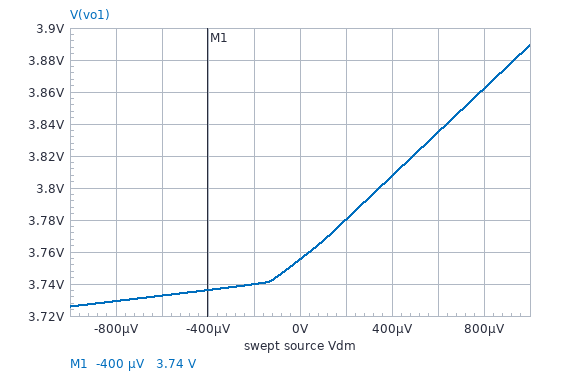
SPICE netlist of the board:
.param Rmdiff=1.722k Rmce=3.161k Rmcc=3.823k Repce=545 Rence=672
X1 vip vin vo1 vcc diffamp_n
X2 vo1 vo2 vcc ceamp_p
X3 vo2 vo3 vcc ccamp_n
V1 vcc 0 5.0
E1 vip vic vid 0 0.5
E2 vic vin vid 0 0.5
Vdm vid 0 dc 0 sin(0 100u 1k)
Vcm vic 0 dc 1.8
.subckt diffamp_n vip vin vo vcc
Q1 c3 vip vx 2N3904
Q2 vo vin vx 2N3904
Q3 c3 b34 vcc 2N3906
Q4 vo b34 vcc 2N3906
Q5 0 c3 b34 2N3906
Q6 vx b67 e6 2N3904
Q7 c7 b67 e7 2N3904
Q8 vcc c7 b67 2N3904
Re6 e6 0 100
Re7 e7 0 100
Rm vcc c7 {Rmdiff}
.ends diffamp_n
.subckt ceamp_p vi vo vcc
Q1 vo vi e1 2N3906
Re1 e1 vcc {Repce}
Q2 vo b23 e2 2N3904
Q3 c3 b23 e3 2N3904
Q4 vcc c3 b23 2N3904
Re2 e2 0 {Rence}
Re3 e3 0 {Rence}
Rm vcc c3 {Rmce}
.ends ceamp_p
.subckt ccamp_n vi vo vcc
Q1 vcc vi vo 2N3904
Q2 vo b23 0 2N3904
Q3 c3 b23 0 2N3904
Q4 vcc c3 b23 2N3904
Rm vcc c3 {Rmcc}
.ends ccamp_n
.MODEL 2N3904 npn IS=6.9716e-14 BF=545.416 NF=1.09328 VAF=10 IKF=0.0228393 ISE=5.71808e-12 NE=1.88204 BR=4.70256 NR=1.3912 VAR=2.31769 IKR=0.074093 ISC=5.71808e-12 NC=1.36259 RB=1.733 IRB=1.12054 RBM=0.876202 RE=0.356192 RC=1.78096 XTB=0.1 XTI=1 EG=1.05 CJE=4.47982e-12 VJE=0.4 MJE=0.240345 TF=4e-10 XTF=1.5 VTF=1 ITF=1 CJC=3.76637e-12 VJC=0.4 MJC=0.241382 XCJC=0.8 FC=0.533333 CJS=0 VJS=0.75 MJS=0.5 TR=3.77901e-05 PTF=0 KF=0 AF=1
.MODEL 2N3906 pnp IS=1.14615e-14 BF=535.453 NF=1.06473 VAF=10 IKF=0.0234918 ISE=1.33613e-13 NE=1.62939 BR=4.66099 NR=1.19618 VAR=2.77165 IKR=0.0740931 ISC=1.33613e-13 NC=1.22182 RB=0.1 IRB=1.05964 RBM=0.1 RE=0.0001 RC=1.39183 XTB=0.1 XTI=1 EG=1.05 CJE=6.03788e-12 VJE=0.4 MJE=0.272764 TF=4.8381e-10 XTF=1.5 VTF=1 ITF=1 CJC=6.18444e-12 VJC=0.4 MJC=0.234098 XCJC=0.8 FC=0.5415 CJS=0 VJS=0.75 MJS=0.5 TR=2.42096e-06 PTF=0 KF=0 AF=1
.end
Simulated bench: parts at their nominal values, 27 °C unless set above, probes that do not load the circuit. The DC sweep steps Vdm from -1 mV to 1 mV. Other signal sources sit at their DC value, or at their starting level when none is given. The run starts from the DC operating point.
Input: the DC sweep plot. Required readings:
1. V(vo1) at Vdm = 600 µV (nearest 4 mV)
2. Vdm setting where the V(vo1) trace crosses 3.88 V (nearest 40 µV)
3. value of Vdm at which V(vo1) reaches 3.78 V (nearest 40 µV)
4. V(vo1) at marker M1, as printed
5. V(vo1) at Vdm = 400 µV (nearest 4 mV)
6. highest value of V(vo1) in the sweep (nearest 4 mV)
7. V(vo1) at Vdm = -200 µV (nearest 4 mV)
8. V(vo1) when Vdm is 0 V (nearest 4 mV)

3.836 V
920 µV
200 µV
3.74 V
3.808 V
3.888 V
3.740 V
3.756 V
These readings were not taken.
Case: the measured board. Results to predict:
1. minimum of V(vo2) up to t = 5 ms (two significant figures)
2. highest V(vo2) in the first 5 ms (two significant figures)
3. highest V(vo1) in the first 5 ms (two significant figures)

1.0 V
3.8 V
3.8 V
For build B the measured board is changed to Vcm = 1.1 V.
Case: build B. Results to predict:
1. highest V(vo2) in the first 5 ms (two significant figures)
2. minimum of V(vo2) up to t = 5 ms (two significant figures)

3.7 V
900 mV
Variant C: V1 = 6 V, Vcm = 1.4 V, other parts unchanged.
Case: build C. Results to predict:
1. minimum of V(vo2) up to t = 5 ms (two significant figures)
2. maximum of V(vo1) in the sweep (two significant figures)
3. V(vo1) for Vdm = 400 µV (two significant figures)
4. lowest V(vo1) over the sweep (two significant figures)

890 mV
4.9 V
4.8 V
4.6 V
